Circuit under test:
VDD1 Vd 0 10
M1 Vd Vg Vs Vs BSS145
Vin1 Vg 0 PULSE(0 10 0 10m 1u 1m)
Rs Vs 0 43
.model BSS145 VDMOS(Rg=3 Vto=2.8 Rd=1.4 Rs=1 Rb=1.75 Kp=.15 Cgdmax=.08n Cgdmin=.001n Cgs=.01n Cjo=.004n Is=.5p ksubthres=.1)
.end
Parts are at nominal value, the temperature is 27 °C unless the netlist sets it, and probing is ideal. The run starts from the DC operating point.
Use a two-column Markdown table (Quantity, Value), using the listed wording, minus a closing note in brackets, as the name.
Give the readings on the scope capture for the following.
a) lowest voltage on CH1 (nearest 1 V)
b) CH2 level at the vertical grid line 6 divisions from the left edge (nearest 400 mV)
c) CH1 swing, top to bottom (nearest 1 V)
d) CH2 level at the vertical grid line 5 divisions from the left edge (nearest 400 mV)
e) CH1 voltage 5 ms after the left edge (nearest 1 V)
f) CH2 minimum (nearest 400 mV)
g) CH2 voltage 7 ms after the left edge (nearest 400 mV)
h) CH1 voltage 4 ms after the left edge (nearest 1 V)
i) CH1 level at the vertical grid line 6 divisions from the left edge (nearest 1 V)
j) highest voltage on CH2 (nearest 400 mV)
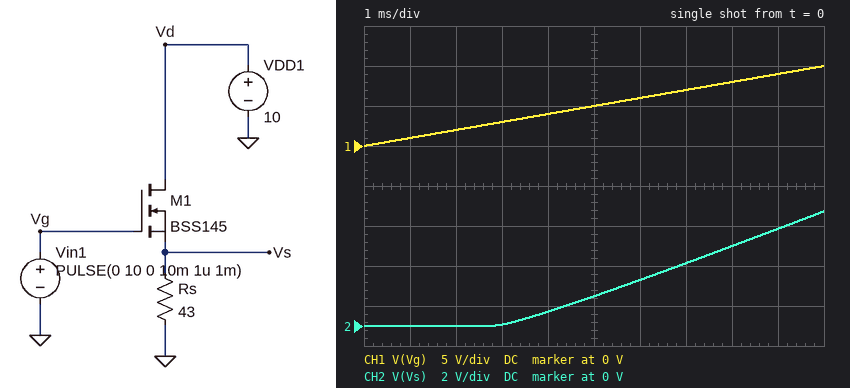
| Quantity | Value |
|---|---|
| lowest voltage on CH1 | 0 V |
| CH2 level at the vertical grid line 6 divisions from the left edge | 2.4 V |
| CH1 swing, top to bottom | 10 V |
| CH2 level at the vertical grid line 5 divisions from the left edge | 1.6 V |
| CH1 voltage 5 ms after the left edge | 5 V |
| CH2 minimum | 0 V |
| CH2 voltage 7 ms after the left edge | 3.2 V |
| CH1 voltage 4 ms after the left edge | 4 V |
| CH1 level at the vertical grid line 6 divisions from the left edge | 6 V |
| highest voltage on CH2 | 5.6 V |
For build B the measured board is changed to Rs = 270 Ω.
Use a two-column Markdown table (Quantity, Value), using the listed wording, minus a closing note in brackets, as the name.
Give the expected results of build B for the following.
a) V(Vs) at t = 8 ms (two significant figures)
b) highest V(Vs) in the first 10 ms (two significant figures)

| Quantity | Value |
|---|---|
| V(Vs) at t = 8 ms | 4.7 V |
| highest V(Vs) in the first 10 ms | 6.6 V |
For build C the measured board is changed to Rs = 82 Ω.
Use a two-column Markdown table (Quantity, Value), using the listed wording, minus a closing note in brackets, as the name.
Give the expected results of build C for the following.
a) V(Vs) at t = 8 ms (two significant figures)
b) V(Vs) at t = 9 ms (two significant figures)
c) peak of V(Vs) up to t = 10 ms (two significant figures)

| Quantity | Value |
|---|---|
| V(Vs) at t = 8 ms | 4.3 V |
| V(Vs) at t = 9 ms | 5.2 V |
| peak of V(Vs) up to t = 10 ms | 6.1 V |
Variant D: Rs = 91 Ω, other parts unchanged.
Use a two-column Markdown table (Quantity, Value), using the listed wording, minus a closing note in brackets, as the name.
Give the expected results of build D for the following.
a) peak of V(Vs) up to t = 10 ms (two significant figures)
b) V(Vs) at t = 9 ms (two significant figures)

| Quantity | Value |
|---|---|
| peak of V(Vs) up to t = 10 ms | 6.2 V |
| V(Vs) at t = 9 ms | 5.3 V |
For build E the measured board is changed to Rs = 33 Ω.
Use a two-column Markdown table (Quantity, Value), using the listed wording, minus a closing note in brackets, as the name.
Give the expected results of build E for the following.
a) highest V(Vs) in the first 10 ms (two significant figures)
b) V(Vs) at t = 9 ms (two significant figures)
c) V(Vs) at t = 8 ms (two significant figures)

| Quantity | Value |
|---|---|
| highest V(Vs) in the first 10 ms | 5.5 V |
| V(Vs) at t = 9 ms | 4.7 V |
| V(Vs) at t = 8 ms | 3.8 V |
